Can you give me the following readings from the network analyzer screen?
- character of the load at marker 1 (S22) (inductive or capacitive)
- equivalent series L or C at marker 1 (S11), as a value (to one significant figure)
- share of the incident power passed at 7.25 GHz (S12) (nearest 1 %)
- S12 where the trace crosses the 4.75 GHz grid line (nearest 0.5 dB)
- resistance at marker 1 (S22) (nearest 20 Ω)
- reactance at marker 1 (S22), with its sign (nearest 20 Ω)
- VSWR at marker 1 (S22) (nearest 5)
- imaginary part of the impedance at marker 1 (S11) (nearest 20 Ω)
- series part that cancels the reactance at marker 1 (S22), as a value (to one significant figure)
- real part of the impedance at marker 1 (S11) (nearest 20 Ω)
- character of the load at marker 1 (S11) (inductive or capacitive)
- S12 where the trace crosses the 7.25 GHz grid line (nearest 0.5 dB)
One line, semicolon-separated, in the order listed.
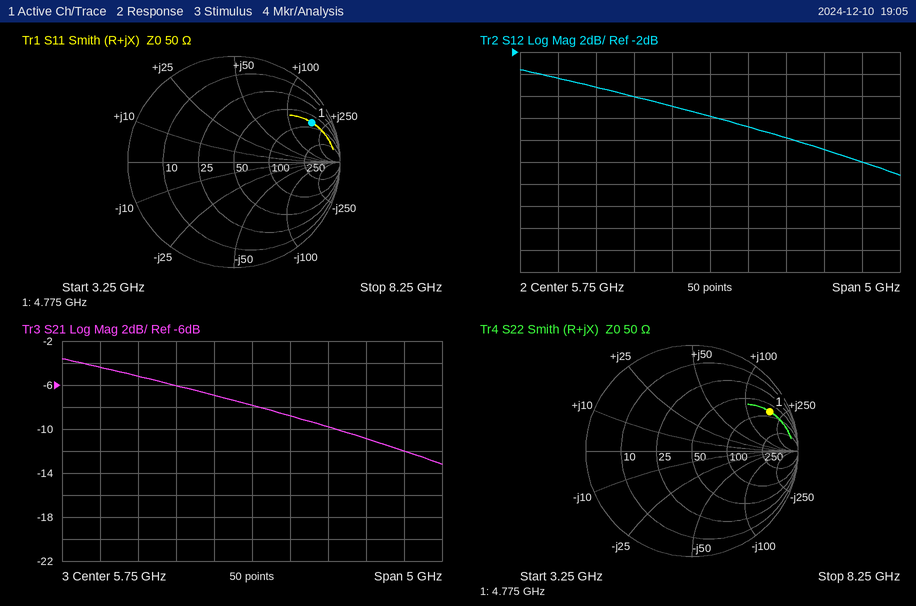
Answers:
inductive; 6 nH; 8 %; -6.0 dB; 80 Ω; +180 Ω; 10; +180 Ω; 200 fF; 80 Ω; inductive; -11.0 dB
